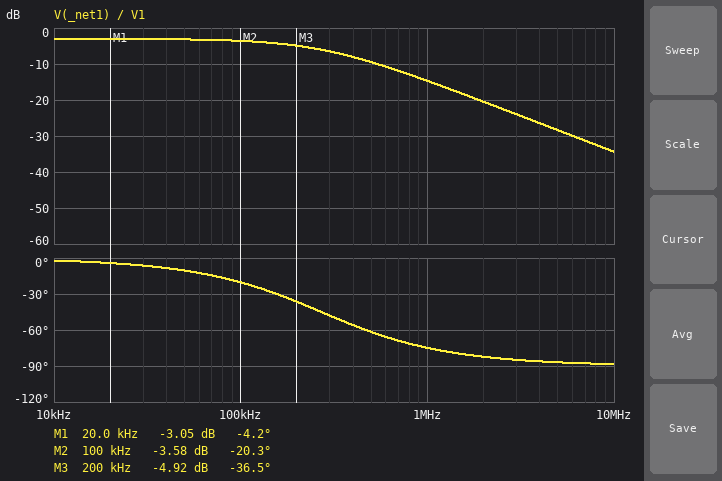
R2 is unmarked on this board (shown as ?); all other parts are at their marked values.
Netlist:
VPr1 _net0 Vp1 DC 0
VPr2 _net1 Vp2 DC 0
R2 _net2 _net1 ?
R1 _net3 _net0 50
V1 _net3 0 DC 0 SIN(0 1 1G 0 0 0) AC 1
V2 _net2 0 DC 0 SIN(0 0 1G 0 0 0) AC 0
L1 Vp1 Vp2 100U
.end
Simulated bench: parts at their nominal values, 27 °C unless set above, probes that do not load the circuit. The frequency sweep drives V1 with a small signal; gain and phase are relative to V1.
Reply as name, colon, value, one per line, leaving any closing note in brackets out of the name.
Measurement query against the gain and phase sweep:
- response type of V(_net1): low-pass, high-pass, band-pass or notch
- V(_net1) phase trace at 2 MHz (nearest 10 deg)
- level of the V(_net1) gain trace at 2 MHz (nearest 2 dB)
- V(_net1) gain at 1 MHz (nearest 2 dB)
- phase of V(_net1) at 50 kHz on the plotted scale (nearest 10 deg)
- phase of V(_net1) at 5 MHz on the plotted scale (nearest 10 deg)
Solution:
response type of V(_net1): low-pass, high-pass, band-pass or notch: low-pass
V(_net1) phase trace at 2 MHz: -80 deg
level of the V(_net1) gain trace at 2 MHz: -20 dB
V(_net1) gain at 1 MHz: -14 dB
phase of V(_net1) at 50 kHz on the plotted scale: -10 deg
phase of V(_net1) at 5 MHz on the plotted scale: -90 deg
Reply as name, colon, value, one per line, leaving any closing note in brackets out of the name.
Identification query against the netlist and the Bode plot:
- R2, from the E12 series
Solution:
R2, from the E12 series: 120 Ω
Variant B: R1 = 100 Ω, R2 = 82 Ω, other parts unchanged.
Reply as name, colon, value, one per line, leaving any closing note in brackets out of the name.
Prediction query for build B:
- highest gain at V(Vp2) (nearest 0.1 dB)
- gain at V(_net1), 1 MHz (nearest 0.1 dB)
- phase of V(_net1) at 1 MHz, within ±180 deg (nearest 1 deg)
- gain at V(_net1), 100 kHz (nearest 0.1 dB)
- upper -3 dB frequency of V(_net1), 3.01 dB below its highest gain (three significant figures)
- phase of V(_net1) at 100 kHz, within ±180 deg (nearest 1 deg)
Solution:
highest gain at V(Vp2): -6.9 dB
gain at V(_net1), 1 MHz: -18.0 dB
phase of V(_net1) at 1 MHz, within ±180 deg: -74 deg
gain at V(_net1), 100 kHz: -7.4 dB
upper -3 dB frequency of V(_net1), 3.01 dB below its highest gain: 290 kHz
phase of V(_net1) at 100 kHz, within ±180 deg: -19 deg
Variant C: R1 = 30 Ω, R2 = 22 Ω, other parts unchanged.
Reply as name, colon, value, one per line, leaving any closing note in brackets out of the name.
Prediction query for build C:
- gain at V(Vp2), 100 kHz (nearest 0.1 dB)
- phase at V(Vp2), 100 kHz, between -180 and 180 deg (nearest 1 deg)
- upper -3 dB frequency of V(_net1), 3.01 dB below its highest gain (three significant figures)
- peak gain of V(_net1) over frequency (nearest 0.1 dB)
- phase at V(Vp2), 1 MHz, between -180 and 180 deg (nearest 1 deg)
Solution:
gain at V(Vp2), 100 kHz: -11.4 dB
phase at V(Vp2), 100 kHz, between -180 and 180 deg: -50 deg
upper -3 dB frequency of V(_net1), 3.01 dB below its highest gain: 82.8 kHz
peak gain of V(_net1) over frequency: -7.5 dB
phase at V(Vp2), 1 MHz, between -180 and 180 deg: -85 deg
